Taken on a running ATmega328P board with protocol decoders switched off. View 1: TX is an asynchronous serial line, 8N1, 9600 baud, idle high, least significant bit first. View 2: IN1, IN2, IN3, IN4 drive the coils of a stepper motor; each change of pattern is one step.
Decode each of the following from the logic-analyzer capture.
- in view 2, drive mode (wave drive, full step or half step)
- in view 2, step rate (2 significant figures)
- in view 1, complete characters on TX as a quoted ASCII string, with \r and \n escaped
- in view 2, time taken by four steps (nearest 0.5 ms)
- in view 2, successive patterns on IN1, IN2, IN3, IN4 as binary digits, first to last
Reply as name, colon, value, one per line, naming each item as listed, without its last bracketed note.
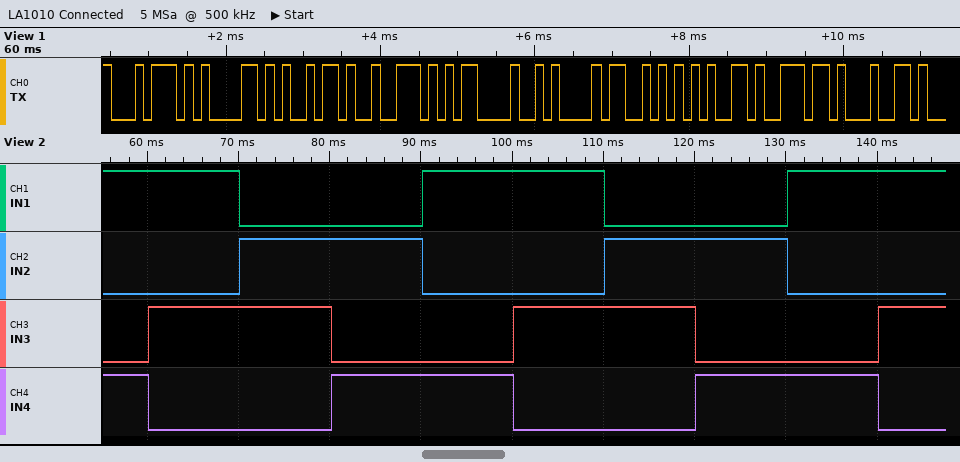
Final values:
in view 2, drive mode: full step
in view 2, step rate: 100 steps/s
in view 1, complete characters on TX as a quoted ASCII string, with \r and \n escaped: "tair\r\nSend"
in view 2, time taken by four steps: 40.0 ms
in view 2, successive patterns on IN1, IN2, IN3, IN4 as binary digits, first to last: 1001 1010 0110 0101 1001 1010 0110 0101 1001 1010
